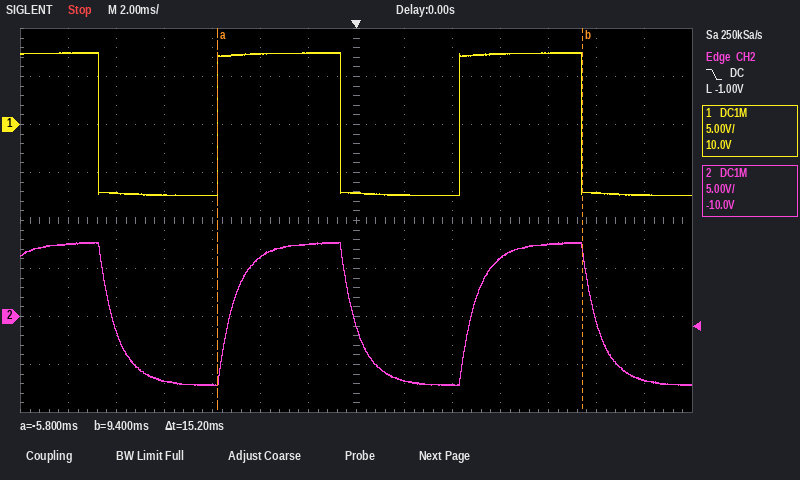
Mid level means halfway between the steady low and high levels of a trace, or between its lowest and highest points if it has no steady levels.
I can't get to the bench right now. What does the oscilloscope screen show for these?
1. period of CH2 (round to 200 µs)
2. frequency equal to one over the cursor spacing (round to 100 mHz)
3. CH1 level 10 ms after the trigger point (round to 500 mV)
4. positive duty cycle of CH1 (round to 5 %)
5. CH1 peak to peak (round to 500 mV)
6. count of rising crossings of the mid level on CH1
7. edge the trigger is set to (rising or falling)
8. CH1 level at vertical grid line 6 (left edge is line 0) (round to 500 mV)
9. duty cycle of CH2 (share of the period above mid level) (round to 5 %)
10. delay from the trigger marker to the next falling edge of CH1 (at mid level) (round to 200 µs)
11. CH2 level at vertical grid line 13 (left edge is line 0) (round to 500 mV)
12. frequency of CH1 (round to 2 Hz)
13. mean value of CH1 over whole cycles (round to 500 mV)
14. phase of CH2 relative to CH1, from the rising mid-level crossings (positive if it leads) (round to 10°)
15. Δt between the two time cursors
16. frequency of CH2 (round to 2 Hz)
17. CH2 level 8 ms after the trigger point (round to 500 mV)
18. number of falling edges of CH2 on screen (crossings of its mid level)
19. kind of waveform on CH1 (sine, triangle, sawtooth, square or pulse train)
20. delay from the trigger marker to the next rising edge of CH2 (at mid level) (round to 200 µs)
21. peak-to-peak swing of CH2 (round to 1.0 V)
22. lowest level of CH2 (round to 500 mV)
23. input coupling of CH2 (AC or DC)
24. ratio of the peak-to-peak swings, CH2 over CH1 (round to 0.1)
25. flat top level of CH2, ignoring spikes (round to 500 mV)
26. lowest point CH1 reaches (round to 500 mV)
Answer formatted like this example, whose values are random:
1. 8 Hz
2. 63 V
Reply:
1. 10.0 ms
2. 65.8 Hz
3. -7.0 V
4. 50 %
5. 15.0 V
6. 2
7. falling
8. 7.5 V
9. 50 %
10. 9.4 ms
11. -6.5 V
12. 100 Hz
13. 0.0 V
14. -20°
15. 15.2 ms
16. 100 Hz
17. 7.5 V
18. 3
19. square
20. 4.8 ms
21. 15.0 V
22. -7.0 V
23. DC
24. 1.0
25. 7.5 V
26. -7.5 V
